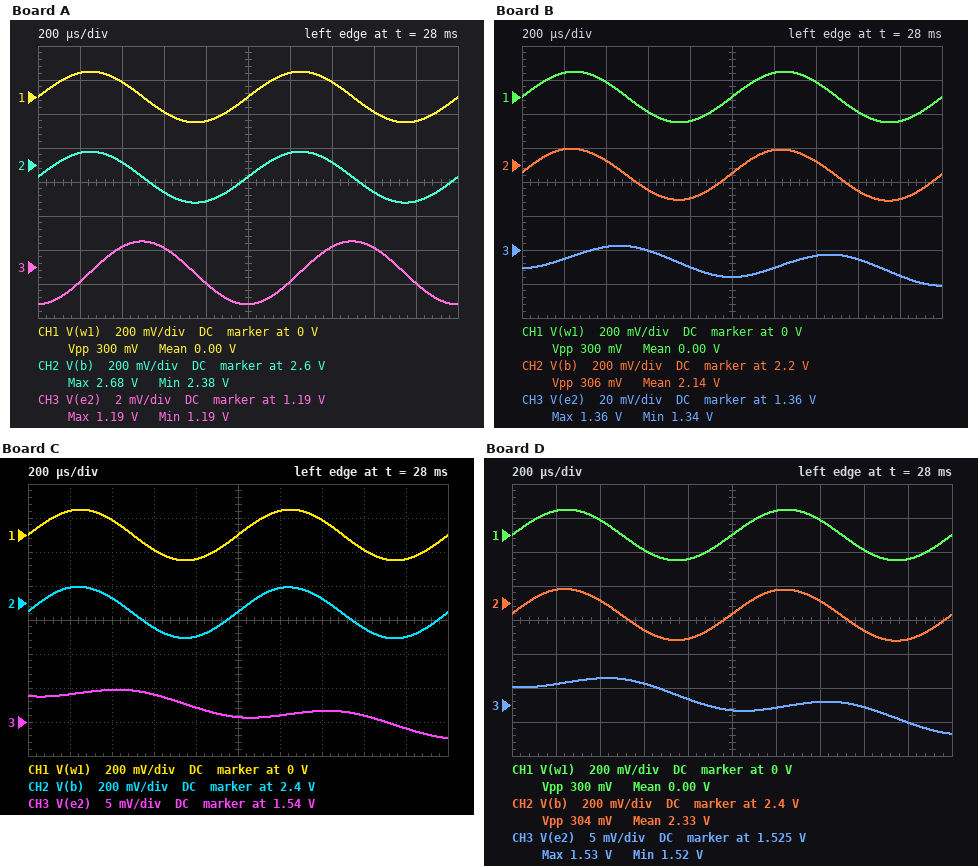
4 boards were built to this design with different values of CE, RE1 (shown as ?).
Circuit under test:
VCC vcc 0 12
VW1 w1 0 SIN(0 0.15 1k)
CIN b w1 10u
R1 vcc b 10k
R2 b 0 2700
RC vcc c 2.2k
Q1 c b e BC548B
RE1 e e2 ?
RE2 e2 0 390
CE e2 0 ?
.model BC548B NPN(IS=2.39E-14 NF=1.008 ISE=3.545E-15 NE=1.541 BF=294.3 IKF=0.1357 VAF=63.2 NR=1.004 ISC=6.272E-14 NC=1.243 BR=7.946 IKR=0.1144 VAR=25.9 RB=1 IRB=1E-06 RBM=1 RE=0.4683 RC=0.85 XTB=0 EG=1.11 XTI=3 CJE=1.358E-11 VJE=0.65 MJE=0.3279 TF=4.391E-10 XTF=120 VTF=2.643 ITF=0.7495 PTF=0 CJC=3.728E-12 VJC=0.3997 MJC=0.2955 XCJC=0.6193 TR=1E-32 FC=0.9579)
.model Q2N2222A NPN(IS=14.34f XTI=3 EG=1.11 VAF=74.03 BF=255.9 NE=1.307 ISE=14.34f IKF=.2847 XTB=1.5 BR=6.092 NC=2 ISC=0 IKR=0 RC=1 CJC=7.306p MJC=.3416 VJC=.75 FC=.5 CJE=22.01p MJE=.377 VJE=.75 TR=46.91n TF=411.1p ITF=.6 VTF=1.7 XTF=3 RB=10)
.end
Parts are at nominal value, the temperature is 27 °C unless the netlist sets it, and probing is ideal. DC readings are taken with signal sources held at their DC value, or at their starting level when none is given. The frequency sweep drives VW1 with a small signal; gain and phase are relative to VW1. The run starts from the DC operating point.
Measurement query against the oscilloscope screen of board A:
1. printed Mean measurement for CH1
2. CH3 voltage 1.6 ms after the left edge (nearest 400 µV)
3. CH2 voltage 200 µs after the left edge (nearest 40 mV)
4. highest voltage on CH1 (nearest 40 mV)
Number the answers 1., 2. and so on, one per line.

1. 0.00 V
2. 1.1912 V
3. 2.68 V
4. 160 mV
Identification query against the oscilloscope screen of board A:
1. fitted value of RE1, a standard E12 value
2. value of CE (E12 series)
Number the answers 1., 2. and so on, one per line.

1. 220 Ω
2. 56 µF
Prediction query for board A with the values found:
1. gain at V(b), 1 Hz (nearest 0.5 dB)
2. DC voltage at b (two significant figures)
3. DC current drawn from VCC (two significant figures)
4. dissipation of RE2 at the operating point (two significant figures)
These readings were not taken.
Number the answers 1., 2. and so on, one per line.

1. -17.5 dB
2. 2.5 V
3. 4.0 mA
4. 3.6 mW
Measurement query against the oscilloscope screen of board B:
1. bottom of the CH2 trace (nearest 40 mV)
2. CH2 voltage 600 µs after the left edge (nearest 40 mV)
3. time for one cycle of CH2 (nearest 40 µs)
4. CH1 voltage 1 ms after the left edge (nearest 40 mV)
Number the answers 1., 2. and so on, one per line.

1. 2.00 V
2. 2.04 V
3. 1.00 ms
4. 0 V
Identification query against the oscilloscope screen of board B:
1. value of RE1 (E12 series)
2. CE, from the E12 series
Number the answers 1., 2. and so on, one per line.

1. 39 Ω
2. 56 µF
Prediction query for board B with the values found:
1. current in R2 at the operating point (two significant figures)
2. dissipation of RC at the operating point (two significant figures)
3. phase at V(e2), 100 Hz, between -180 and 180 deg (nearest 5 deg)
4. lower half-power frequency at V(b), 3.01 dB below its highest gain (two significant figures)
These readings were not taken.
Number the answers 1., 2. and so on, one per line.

1. 930 µA
2. 40 mW
3. -50 deg
4. 7.8 Hz
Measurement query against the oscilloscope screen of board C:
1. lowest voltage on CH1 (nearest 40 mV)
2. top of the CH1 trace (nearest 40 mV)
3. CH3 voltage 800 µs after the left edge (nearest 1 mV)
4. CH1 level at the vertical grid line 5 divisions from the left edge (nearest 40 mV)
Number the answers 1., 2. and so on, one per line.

1. -160 mV
2. 160 mV
3. 1.542 V
4. 0 V
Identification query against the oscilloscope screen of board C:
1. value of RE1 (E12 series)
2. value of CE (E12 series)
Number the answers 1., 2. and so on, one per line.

1. 47 Ω
2. 330 µF
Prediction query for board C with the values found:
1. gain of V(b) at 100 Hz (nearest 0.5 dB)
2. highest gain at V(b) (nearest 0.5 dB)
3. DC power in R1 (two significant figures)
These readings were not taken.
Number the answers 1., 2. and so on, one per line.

1. 0 dB
2. 0 dB
3. 9.0 mW
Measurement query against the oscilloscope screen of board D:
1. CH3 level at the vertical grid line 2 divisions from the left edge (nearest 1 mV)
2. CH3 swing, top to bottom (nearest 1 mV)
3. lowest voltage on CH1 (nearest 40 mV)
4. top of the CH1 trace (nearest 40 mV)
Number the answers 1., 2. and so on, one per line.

1. 1.529 V
2. 8 mV
3. -160 mV
4. 160 mV
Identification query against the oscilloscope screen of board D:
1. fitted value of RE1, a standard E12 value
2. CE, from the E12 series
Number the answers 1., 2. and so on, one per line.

1. 47 Ω
2. 270 µF
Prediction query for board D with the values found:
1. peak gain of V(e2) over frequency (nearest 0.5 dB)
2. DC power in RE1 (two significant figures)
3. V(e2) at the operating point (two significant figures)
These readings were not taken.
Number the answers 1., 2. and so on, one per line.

1. -6.0 dB
2. 830 µW
3. 1.6 V
